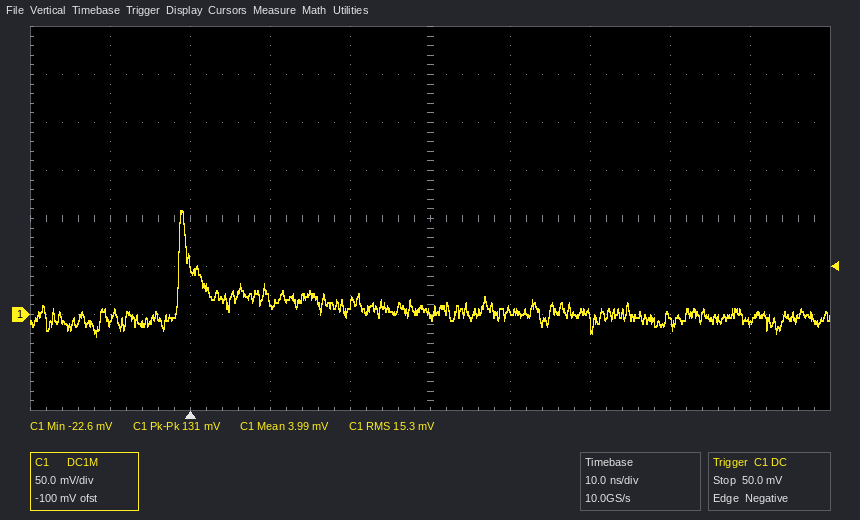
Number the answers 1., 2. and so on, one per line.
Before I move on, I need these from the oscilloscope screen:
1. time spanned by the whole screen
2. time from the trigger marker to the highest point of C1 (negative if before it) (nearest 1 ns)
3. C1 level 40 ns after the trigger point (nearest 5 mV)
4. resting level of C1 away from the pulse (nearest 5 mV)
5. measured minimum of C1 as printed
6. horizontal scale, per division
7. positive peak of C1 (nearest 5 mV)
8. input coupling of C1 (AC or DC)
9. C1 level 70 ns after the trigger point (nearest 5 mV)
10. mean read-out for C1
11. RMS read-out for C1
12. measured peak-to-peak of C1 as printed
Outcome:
1. 100 ns
2. -1 ns
3. 5 mV
4. 0 mV
5. -22.6 mV
6. 10 ns
7. 110 mV
8. DC
9. -10 mV
10. 3.99 mV
11. 15.3 mV
12. 131 mV
